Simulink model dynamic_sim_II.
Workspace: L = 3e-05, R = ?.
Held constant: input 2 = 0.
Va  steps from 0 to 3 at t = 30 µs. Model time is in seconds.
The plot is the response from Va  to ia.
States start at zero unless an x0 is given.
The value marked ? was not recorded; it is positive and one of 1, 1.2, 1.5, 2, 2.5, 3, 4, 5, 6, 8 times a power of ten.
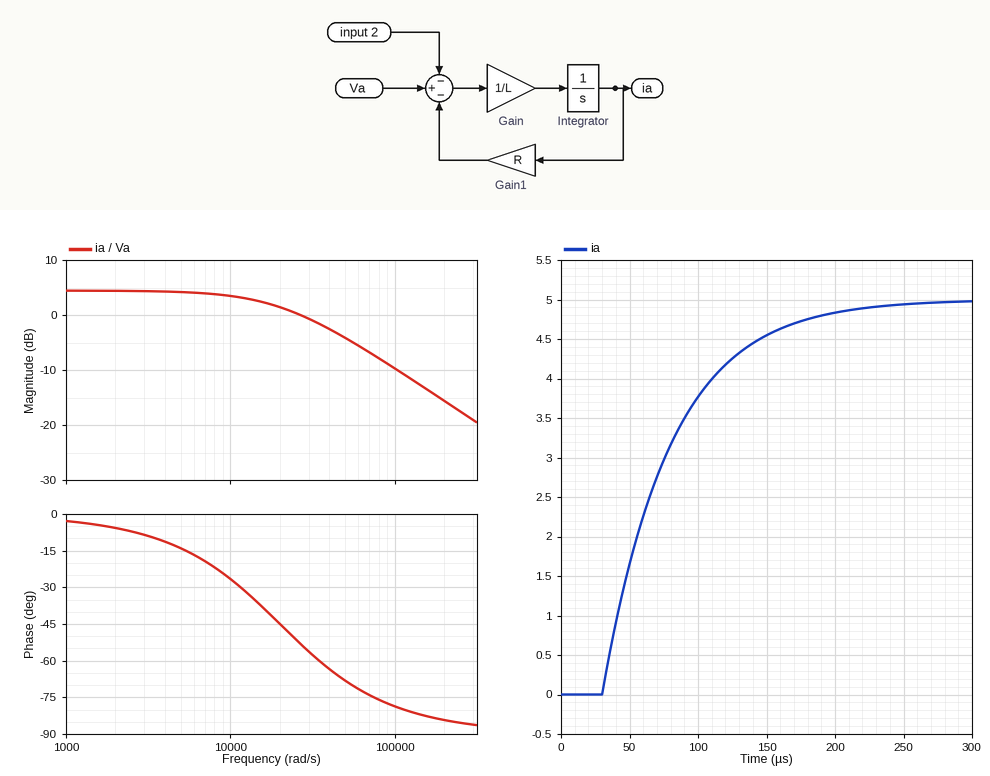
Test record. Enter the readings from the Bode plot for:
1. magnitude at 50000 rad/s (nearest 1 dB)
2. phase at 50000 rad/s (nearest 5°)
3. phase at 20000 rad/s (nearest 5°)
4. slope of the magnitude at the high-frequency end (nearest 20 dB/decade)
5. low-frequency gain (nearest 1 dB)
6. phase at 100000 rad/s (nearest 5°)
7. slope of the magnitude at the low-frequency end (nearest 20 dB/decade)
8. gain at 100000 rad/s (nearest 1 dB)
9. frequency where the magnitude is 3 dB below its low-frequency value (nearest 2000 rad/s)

-4 dB
-70°
-45°
-20 dB/decade
4 dB
-80°
0 dB/decade
-10 dB
20000 rad/s
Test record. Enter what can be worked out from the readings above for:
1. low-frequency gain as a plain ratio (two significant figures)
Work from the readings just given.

1.6
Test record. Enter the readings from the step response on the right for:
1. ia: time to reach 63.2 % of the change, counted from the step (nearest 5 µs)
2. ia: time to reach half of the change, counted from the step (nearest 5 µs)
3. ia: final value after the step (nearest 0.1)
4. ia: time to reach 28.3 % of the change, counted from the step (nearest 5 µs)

50 µs
35 µs
5.0
15 µs
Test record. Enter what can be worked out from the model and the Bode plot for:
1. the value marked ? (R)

0.6
